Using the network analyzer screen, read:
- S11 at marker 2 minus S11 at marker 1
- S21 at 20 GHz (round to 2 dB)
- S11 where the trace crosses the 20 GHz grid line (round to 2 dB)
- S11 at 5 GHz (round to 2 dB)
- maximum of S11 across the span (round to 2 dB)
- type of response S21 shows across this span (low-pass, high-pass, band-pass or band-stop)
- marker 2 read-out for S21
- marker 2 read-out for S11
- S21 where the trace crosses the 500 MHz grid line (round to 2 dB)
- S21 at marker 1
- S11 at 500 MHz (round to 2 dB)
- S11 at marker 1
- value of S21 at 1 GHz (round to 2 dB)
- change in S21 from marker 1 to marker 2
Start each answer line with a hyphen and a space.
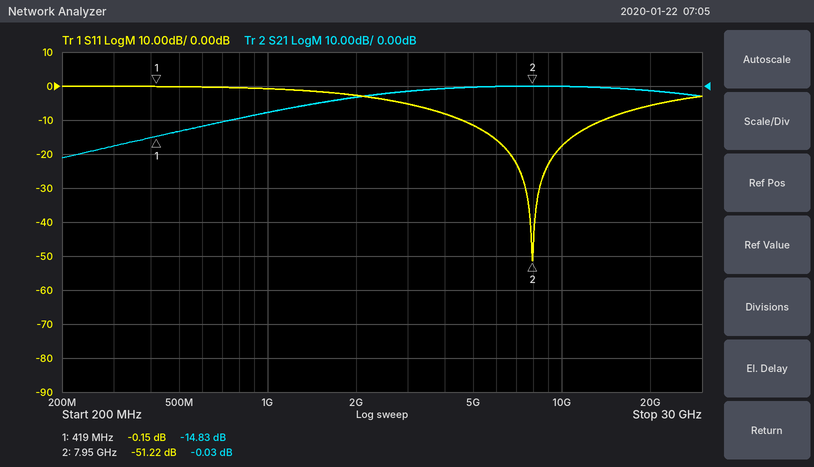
- -51.07 dB
- -2 dB
- -6 dB
- -12 dB
- 0 dB
- high-pass
- -0.03 dB
- -51.22 dB
- -14 dB
- -14.83 dB
- 0 dB
- -0.15 dB
- -8 dB
- 14.80 dB
